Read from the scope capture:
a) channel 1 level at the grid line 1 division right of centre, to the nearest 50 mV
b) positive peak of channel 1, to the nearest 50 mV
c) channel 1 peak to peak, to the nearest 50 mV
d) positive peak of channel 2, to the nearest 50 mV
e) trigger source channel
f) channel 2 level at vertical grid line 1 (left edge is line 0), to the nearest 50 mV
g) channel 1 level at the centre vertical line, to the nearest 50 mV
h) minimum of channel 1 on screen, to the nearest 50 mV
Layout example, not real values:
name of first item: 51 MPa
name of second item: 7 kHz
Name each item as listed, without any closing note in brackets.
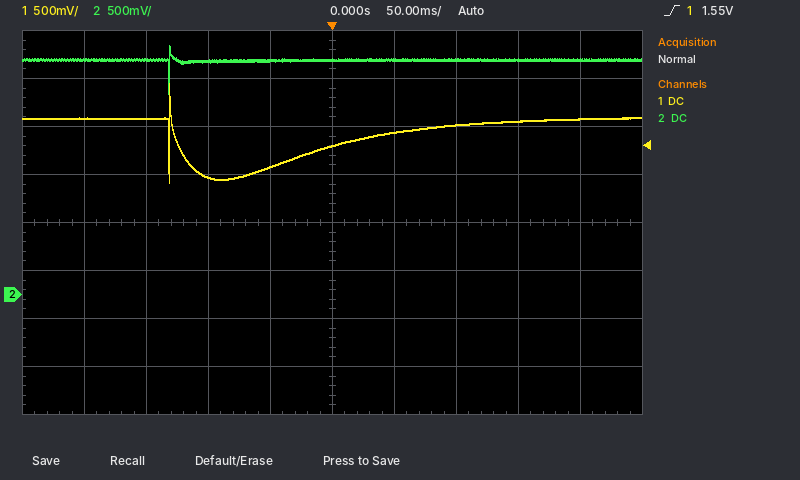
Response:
channel 1 level at the grid line 1 division right of centre, to the nearest 50 mV: 1.70 V
positive peak of channel 1, to the nearest 50 mV: 2.20 V
channel 1 peak to peak, to the nearest 50 mV: 1.05 V
positive peak of channel 2, to the nearest 50 mV: 2.60 V
trigger source channel: channel 1
channel 2 level at vertical grid line 1 (left edge is line 0), to the nearest 50 mV: 2.45 V
channel 1 level at the centre vertical line, to the nearest 50 mV: 1.55 V
minimum of channel 1 on screen, to the nearest 50 mV: 1.15 V
